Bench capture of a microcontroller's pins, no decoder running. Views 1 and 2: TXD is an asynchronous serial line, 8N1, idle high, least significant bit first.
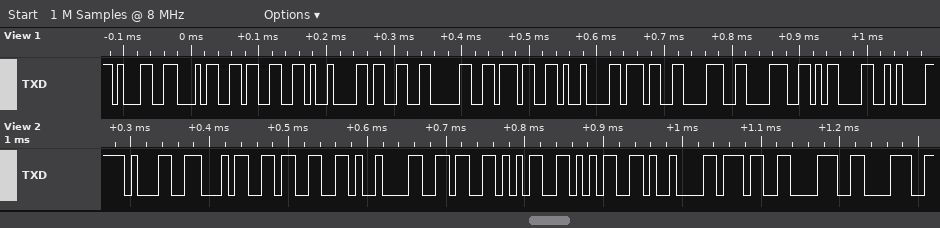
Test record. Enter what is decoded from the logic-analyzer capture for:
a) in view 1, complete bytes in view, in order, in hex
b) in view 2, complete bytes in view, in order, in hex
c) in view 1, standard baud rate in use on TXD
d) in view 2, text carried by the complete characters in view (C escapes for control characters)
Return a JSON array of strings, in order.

["31 34 33 09 33 30 37 09 37 38 38 0D 0A", "0x31 0x34 0x33 0x09 0x36 0x35 0x35 0x09 0x37 0x38 0x38", "115200 baud", "\"143\\t655\\t788\""]
